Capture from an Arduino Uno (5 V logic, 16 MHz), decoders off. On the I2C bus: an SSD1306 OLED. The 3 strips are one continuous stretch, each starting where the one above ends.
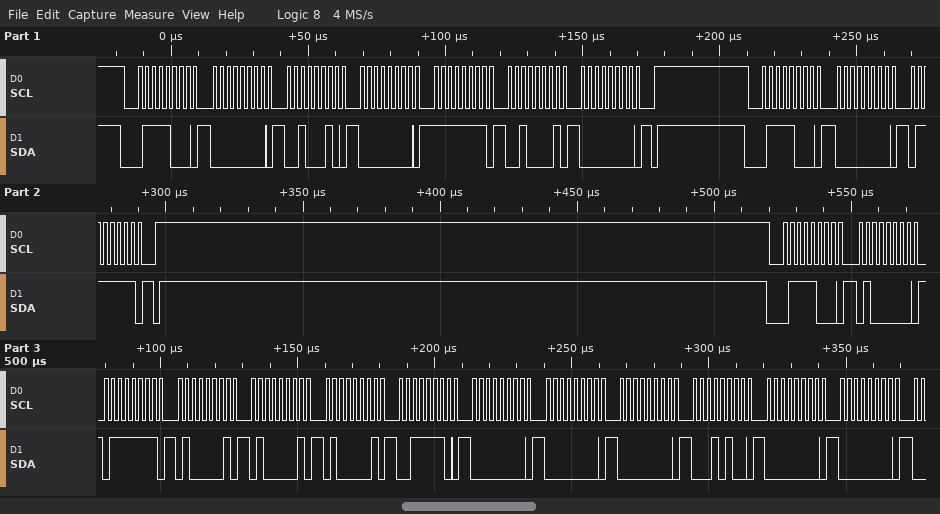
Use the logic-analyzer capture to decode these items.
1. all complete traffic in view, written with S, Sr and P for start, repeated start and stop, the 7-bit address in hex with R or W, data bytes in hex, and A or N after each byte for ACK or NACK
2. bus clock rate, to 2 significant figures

S 3CW A 00 A 22 A 00 A FF A 21 A 00 A P S 3CW A 00 A 7F A P S 3CW A 40 A 7F A 41 A 41 A 41 A 3E A 00 A 00 A 00 A 14 A 00 A 00 A
400 kHz
